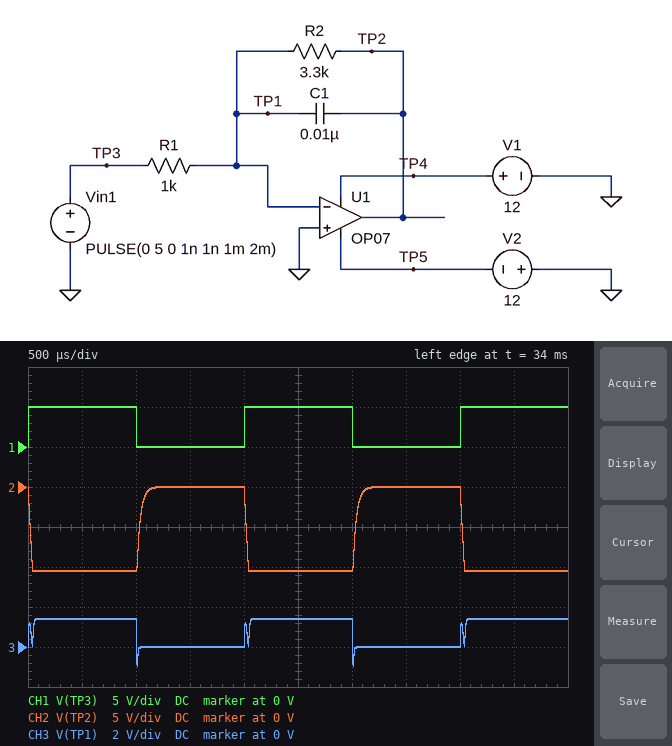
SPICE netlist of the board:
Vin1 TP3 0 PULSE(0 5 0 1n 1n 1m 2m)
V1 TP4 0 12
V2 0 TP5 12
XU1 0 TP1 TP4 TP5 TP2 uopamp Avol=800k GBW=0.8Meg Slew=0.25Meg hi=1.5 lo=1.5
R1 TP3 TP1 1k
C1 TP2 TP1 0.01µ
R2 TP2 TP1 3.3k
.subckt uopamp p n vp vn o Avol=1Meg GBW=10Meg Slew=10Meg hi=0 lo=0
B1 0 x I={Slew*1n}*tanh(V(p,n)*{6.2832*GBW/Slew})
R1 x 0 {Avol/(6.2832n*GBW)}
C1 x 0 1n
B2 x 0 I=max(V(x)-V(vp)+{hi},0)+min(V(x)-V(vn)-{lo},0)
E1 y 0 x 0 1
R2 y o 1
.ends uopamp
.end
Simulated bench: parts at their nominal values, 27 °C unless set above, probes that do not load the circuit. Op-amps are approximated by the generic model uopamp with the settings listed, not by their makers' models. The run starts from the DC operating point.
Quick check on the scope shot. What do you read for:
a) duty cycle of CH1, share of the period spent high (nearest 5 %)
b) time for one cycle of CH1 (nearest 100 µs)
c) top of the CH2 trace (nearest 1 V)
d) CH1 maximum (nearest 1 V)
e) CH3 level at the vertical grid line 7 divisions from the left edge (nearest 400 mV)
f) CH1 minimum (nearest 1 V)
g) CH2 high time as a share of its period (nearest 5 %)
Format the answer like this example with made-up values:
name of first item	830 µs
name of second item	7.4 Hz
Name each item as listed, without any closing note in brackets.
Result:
duty cycle of CH1, share of the period spent high	50 %
time for one cycle of CH1	2.0 ms
top of the CH2 trace	0 V
CH1 maximum	5 V
CH3 level at the vertical grid line 7 divisions from the left edge	0 V
CH1 minimum	0 V
CH2 high time as a share of its period	50 %
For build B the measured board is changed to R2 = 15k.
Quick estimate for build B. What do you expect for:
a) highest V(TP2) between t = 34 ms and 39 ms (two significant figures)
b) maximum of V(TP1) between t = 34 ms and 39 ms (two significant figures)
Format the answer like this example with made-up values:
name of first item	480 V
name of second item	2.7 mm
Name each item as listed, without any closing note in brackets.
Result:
highest V(TP2) between t = 34 ms and 39 ms	-12 mV
maximum of V(TP1) between t = 34 ms and 39 ms	4.0 V
